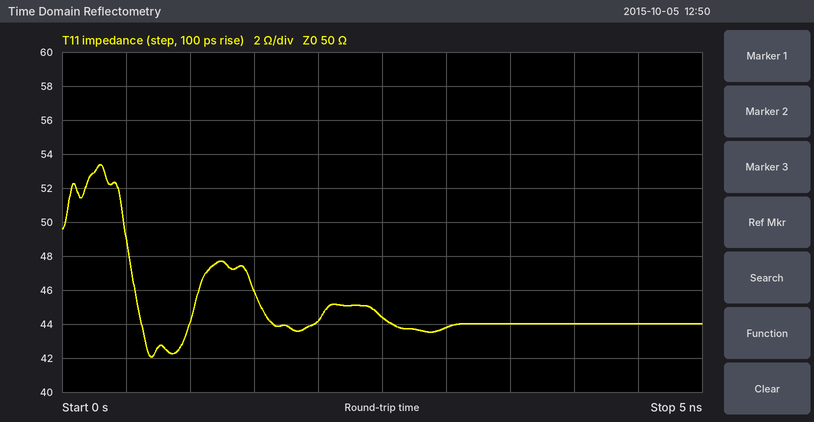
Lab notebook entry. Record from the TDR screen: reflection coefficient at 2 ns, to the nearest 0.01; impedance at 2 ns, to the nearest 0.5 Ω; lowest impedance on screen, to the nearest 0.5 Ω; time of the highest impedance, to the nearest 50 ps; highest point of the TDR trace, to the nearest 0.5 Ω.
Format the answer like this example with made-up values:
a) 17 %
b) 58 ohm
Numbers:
a) -0.06
b) 44.0 Ω
c) 42.0 Ω
d) 300 ps
e) 53.5 Ω
